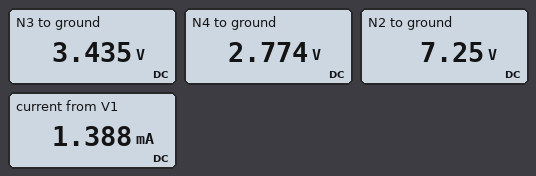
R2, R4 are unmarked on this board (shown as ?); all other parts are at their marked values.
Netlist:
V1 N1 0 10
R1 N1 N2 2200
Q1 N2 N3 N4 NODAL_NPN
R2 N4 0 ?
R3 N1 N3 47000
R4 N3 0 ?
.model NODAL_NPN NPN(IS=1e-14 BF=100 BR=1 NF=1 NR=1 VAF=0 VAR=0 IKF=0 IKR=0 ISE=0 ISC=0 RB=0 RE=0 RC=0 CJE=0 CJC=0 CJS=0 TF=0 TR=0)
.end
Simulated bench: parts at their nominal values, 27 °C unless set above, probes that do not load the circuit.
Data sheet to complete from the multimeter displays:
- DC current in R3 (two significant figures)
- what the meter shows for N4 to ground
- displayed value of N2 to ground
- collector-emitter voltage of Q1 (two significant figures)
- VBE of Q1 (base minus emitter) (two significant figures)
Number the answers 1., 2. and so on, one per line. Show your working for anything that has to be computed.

1. (10 V - 3.435 V) / 47 kΩ = 140 µA
2. 2.774 V
3. 7.25 V
4. 7.25 V - 2.774 V = 4.5 V
5. 3.435 V - 2.774 V = 660 mV
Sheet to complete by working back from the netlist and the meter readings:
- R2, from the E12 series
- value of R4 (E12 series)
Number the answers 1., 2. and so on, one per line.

1. 2.2 kΩ
2. 27 kΩ
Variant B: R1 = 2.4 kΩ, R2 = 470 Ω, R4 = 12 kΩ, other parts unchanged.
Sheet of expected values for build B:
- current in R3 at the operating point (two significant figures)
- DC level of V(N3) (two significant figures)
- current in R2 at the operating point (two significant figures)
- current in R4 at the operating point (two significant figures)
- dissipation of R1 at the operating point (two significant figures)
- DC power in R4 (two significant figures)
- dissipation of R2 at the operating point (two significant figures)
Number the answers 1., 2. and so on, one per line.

1. 170 µA
2. 1.8 V
3. 2.4 mA
4. 150 µA
5. 14 mW
6. 270 µW
7. 2.7 mW
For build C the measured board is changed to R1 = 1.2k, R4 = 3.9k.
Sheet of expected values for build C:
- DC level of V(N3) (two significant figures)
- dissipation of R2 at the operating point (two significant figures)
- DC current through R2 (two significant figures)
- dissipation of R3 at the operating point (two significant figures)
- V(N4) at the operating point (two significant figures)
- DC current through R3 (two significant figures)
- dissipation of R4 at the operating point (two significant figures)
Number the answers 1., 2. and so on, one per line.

1. 760 mV
2. 14 µW
3. 79 µA
4. 1.8 mW
5. 170 mV
6. 200 µA
7. 150 µW
